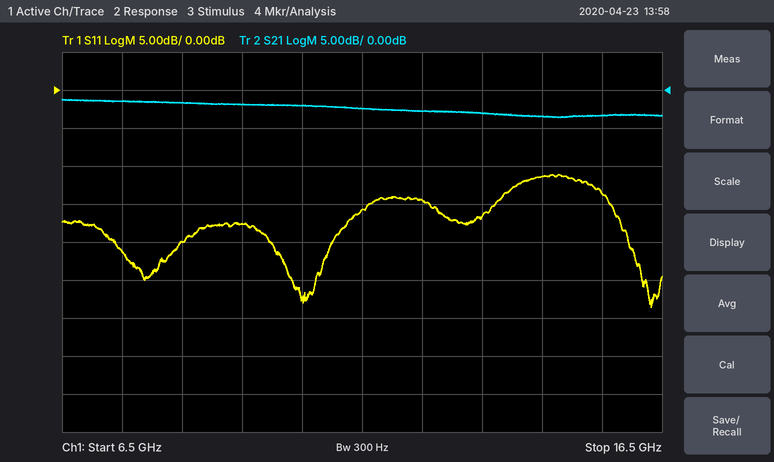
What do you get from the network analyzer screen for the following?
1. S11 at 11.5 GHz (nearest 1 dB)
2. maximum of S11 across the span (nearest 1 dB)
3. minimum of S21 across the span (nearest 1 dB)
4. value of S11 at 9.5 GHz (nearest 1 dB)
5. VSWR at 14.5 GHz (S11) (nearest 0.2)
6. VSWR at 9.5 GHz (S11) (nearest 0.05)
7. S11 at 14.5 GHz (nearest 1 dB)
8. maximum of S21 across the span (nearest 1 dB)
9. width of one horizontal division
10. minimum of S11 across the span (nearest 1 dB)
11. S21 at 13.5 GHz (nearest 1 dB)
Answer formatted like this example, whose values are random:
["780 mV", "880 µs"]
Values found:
["-16 dB", "-11 dB", "-4 dB", "-18 dB", "1.8", "1.30", "-11 dB", "-1 dB", "1 GHz", "-29 dB", "-3 dB"]
